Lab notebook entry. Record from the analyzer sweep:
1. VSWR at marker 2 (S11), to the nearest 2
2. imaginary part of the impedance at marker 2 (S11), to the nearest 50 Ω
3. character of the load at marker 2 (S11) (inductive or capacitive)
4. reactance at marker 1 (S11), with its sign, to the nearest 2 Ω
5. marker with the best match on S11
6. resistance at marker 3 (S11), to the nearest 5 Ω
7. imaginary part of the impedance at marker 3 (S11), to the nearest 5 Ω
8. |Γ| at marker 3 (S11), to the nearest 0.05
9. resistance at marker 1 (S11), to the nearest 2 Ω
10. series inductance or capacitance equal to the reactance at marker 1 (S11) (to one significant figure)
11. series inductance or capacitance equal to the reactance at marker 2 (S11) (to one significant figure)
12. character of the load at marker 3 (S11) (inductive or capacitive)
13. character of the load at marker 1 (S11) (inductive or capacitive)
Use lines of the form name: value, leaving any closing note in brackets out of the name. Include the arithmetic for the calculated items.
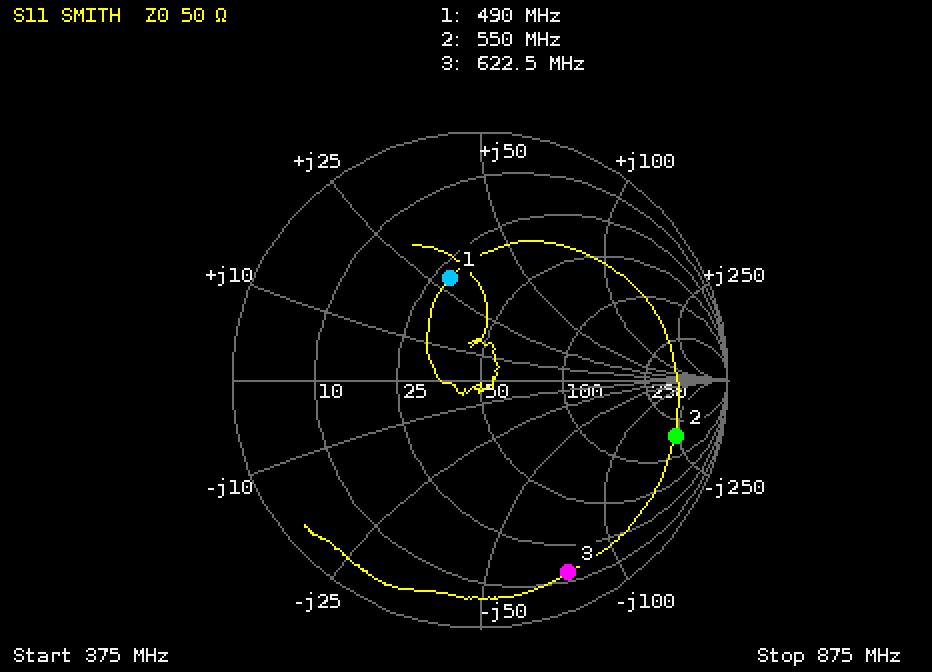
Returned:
VSWR at marker 2 (S11), to the nearest 2: 10
imaginary part of the impedance at marker 2 (S11), to the nearest 50 Ω: -250 Ω
character of the load at marker 2 (S11): capacitive
reactance at marker 1 (S11), with its sign, to the nearest 2 Ω: +28 Ω
marker with the best match on S11: marker 1
resistance at marker 3 (S11), to the nearest 5 Ω: 15 Ω
imaginary part of the impedance at marker 3 (S11), to the nearest 5 Ω: -75 Ω
|Γ| at marker 3 (S11), to the nearest 0.05: 0.85
resistance at marker 1 (S11), to the nearest 2 Ω: 28 Ω
series inductance or capacitance equal to the reactance at marker 1 (S11): L = 28 Ω/(2π × 490 MHz) ≈ 9 nH
series inductance or capacitance equal to the reactance at marker 2 (S11): C = 1/(2π × 550 MHz × 250 Ω) ≈ 1 pF
character of the load at marker 3 (S11): capacitive
character of the load at marker 1 (S11): inductive
